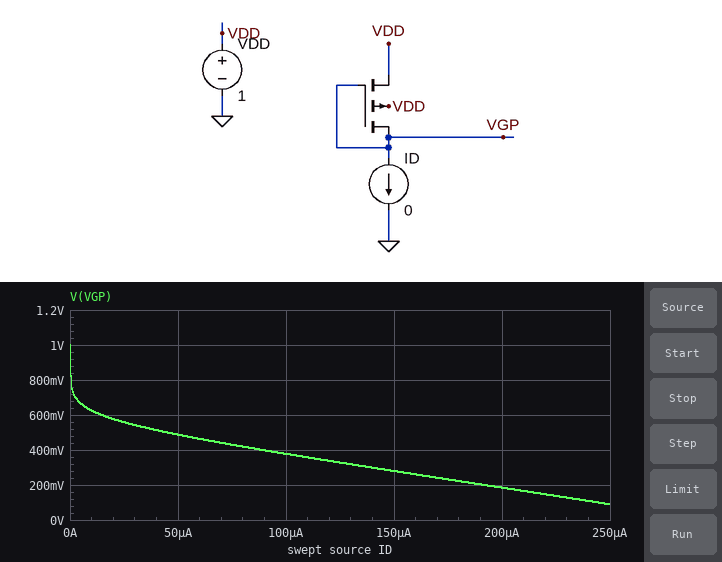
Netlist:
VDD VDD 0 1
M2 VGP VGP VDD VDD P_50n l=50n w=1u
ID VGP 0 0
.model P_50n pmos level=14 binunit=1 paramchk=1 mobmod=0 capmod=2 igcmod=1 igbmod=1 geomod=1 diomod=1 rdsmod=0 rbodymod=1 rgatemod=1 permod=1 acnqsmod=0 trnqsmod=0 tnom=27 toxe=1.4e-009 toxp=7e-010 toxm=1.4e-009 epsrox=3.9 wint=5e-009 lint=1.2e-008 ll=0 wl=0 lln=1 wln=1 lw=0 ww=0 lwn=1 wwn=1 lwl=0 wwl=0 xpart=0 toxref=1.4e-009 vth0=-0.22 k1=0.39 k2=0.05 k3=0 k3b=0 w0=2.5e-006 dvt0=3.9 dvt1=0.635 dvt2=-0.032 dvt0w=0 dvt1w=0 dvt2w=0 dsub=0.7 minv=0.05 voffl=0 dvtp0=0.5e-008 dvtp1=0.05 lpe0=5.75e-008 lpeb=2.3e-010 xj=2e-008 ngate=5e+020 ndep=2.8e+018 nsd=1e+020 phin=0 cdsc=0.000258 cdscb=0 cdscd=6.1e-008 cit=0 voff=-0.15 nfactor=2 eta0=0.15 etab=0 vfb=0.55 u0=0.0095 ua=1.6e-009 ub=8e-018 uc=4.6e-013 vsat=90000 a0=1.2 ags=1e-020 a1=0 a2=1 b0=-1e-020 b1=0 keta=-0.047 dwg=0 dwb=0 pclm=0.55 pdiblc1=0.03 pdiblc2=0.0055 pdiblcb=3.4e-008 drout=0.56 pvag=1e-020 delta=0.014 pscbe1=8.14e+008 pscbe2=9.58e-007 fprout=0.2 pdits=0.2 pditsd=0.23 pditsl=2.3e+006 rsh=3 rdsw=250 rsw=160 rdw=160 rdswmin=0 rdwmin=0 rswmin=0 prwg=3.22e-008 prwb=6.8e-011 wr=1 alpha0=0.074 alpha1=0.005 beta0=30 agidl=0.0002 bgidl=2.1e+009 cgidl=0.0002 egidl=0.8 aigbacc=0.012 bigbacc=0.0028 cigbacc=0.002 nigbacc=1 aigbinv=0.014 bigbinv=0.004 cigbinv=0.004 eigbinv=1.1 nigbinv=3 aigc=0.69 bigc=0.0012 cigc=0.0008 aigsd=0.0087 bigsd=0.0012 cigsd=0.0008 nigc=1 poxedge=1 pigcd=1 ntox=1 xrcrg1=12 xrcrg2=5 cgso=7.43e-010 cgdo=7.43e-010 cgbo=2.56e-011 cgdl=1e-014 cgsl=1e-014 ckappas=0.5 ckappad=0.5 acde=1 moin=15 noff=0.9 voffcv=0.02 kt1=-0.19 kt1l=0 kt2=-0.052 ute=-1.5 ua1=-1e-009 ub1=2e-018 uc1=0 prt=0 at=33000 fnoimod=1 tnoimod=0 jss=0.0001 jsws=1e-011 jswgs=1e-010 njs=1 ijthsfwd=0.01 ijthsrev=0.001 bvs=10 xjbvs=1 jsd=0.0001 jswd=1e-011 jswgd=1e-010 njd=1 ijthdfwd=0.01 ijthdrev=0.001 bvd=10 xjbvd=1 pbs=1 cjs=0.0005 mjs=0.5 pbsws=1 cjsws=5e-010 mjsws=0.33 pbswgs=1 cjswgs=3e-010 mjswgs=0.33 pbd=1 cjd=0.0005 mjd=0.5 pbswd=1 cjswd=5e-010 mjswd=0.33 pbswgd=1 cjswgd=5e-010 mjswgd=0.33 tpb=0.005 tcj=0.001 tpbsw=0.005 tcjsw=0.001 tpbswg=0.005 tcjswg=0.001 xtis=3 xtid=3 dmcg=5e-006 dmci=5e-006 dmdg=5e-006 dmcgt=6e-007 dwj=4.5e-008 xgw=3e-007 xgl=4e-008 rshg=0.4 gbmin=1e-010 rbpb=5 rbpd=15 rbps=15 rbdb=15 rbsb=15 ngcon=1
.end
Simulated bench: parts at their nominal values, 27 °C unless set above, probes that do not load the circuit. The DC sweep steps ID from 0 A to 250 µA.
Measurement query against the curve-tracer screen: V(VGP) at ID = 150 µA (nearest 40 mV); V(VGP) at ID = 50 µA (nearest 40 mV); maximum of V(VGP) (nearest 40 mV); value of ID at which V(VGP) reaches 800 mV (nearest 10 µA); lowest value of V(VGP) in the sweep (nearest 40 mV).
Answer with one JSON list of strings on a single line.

["280 mV", "480 mV", "1.00 V", "0 A", "80 mV"]
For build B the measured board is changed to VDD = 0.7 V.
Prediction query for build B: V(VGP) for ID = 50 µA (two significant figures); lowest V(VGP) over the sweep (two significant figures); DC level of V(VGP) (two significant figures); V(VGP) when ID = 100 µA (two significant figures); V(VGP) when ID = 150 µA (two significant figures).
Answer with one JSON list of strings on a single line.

["190 mV", "-210 mV", "700 mV", "78 mV", "-20 mV"]
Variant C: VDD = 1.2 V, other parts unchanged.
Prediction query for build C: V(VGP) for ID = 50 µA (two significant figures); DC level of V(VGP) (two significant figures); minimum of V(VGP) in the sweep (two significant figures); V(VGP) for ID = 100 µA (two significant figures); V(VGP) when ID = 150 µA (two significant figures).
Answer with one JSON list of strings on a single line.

["690 mV", "1.2 V", "290 mV", "580 mV", "480 mV"]
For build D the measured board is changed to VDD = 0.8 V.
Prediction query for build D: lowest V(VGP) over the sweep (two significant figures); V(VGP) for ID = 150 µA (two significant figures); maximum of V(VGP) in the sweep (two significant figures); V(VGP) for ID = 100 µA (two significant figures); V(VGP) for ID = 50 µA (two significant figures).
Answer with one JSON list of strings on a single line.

["-110 mV", "80 mV", "800 mV", "180 mV", "290 mV"]
